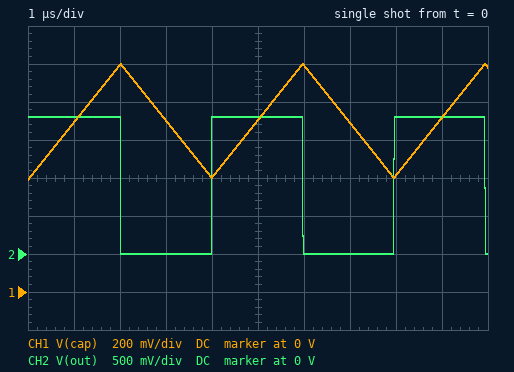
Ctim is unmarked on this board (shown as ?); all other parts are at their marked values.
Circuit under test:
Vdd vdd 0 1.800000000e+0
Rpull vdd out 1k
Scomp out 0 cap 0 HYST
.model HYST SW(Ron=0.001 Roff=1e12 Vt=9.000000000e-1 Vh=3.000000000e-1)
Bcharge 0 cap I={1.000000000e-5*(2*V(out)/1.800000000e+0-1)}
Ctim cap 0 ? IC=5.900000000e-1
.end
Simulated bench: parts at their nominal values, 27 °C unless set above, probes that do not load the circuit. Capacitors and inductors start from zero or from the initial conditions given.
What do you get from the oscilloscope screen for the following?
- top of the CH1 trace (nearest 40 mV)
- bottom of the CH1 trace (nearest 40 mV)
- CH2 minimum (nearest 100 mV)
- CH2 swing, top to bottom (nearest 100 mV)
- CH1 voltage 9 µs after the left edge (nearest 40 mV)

1.20 V
600 mV
0 V
1.8 V
920 mV
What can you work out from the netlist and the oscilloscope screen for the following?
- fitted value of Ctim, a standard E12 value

33 pF
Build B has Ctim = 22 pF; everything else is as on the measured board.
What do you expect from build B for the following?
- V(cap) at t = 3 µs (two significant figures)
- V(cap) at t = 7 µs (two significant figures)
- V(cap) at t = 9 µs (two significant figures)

750 mV
1.0 V
1.1 V
